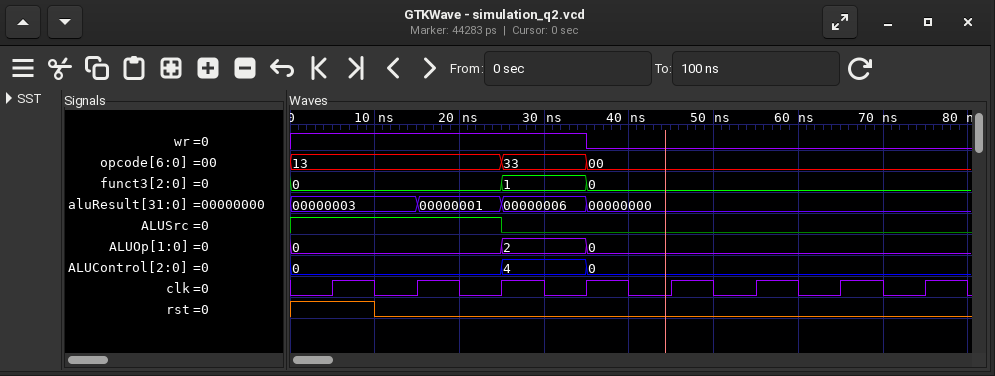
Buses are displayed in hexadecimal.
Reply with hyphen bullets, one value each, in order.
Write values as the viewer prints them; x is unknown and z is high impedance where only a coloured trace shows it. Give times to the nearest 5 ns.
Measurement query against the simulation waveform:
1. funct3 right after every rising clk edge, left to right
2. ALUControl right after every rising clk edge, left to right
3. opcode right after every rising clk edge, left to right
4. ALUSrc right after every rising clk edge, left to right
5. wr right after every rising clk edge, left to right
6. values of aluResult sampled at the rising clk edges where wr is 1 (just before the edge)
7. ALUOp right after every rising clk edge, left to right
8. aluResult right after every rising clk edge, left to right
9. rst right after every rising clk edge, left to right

- 0, 0, 1, 0, 0, 0, 0, 0
- 0, 0, 4, 0, 0, 0, 0, 0
- 13, 13, 33, 00, 00, 00, 00, 00
- 1 1 0 0 0 0 0 0
- 1 1 1 0 0 0 0 0
- 00000003, 00000003, 00000001, 00000006
- 0, 0, 2, 0, 0, 0, 0, 0
- 00000003, 00000001, 00000006, 00000000, 00000000, 00000000, 00000000, 00000000
- 1 0 0 0 0 0 0 0
